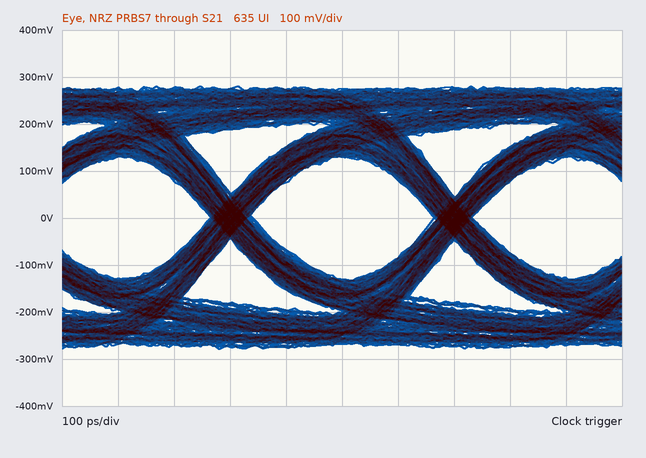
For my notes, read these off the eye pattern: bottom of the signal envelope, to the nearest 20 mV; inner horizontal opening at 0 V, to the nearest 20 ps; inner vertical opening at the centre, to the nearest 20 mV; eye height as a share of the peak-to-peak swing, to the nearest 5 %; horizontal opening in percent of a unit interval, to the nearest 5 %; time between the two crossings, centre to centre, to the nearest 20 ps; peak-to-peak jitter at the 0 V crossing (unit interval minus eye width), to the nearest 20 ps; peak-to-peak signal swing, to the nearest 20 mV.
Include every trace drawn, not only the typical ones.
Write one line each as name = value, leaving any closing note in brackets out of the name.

bottom of the signal envelope, to the nearest 20 mV = -280 mV
inner horizontal opening at 0 V, to the nearest 20 ps = 320 ps
inner vertical opening at the centre, to the nearest 20 mV = 260 mV
eye height as a share of the peak-to-peak swing, to the nearest 5 % = 45 %
horizontal opening in percent of a unit interval, to the nearest 5 % = 80 %
time between the two crossings, centre to centre, to the nearest 20 ps = 400 ps
peak-to-peak jitter at the 0 V crossing (unit interval minus eye width), to the nearest 20 ps = 80 ps
peak-to-peak signal swing, to the nearest 20 mV = 560 mV
